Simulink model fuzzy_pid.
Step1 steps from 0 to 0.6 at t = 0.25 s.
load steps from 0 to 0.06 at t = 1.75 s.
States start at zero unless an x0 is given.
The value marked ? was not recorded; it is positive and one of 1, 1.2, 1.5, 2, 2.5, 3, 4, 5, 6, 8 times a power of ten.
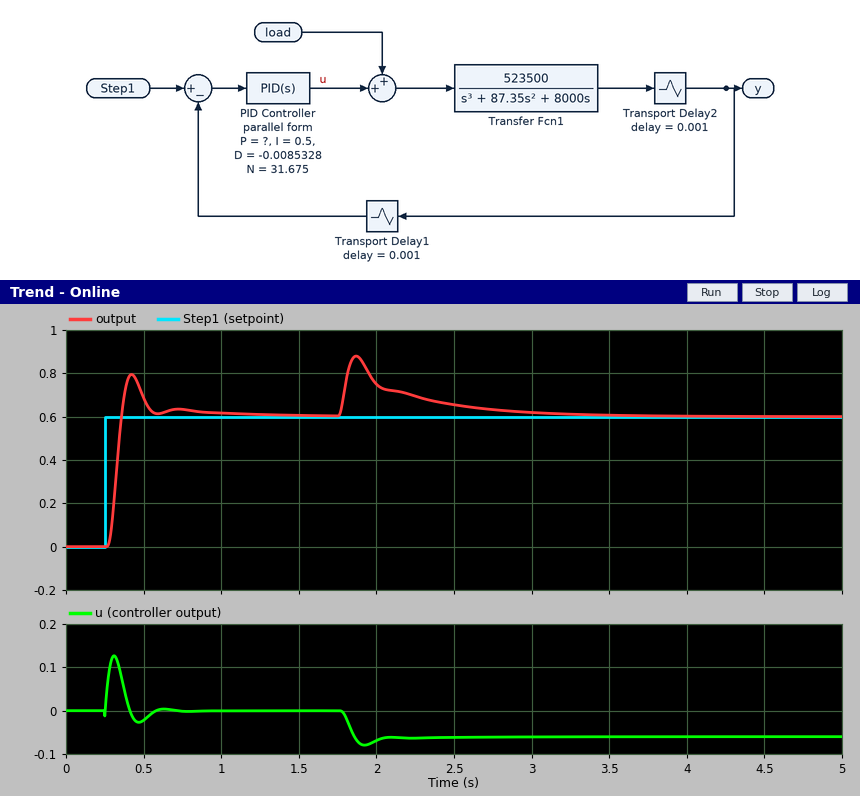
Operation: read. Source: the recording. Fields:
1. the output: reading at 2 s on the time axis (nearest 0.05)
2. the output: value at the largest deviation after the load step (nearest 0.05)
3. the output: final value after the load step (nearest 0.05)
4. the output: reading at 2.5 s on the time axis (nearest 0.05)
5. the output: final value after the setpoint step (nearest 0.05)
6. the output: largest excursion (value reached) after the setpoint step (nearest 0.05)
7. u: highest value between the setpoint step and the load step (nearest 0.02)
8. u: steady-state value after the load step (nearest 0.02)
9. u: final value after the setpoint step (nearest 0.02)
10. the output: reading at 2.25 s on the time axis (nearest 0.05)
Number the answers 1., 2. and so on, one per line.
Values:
1. 0.75
2. 0.90
3. 0.60
4. 0.65
5. 0.60
6. 0.80
7. 0.12
8. -0.06
9. 0.00
10. 0.70
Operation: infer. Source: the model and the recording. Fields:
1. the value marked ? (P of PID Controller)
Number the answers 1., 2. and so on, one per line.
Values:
1. 0.25
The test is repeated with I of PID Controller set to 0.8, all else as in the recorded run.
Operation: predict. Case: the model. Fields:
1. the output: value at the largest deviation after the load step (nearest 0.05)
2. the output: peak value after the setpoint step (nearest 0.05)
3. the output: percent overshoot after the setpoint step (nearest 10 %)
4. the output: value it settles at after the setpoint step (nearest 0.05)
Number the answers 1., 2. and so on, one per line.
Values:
1. 0.85
2. 0.85
3. 40 %
4. 0.60
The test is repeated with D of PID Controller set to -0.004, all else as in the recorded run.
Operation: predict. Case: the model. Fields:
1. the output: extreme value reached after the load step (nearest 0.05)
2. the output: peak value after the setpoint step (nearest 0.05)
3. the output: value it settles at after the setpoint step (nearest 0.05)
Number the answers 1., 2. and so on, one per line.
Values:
1. 0.85
2. 0.70
3. 0.60
